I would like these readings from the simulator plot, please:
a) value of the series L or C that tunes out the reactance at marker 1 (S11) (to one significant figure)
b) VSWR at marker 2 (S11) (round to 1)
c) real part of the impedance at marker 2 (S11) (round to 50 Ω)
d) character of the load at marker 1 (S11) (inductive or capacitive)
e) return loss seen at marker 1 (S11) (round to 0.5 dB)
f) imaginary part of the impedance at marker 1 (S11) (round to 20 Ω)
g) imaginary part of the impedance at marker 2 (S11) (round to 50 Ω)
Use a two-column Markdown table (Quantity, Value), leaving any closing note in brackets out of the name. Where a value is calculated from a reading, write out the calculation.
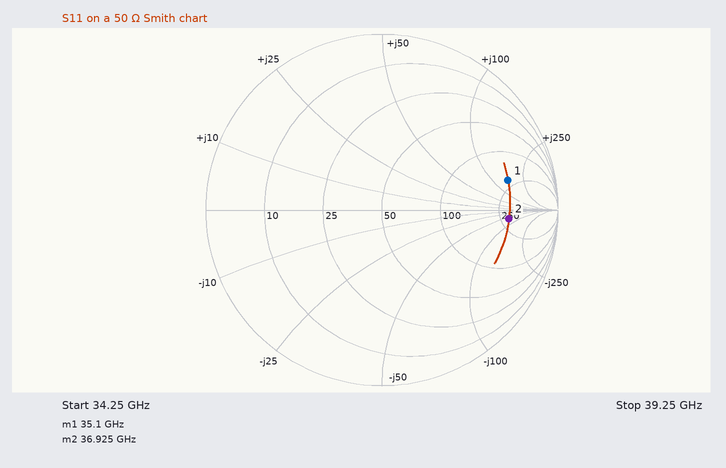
| Quantity | Value |
|---|---|
| value of the series L or C that tunes out the reactance at marker 1 (S11) | C = 1/(2π × 35.1 GHz × 160 Ω) ≈ 28.3 fF, so 30 fF to one significant figure |
| VSWR at marker 2 (S11) | 6 |
| real part of the impedance at marker 2 (S11) | 300 Ω |
| character of the load at marker 1 (S11) | inductive |
| return loss seen at marker 1 (S11) | 2.5 dB |
| imaginary part of the impedance at marker 1 (S11) | +160 Ω |
| imaginary part of the impedance at marker 2 (S11) | -50 Ω |
